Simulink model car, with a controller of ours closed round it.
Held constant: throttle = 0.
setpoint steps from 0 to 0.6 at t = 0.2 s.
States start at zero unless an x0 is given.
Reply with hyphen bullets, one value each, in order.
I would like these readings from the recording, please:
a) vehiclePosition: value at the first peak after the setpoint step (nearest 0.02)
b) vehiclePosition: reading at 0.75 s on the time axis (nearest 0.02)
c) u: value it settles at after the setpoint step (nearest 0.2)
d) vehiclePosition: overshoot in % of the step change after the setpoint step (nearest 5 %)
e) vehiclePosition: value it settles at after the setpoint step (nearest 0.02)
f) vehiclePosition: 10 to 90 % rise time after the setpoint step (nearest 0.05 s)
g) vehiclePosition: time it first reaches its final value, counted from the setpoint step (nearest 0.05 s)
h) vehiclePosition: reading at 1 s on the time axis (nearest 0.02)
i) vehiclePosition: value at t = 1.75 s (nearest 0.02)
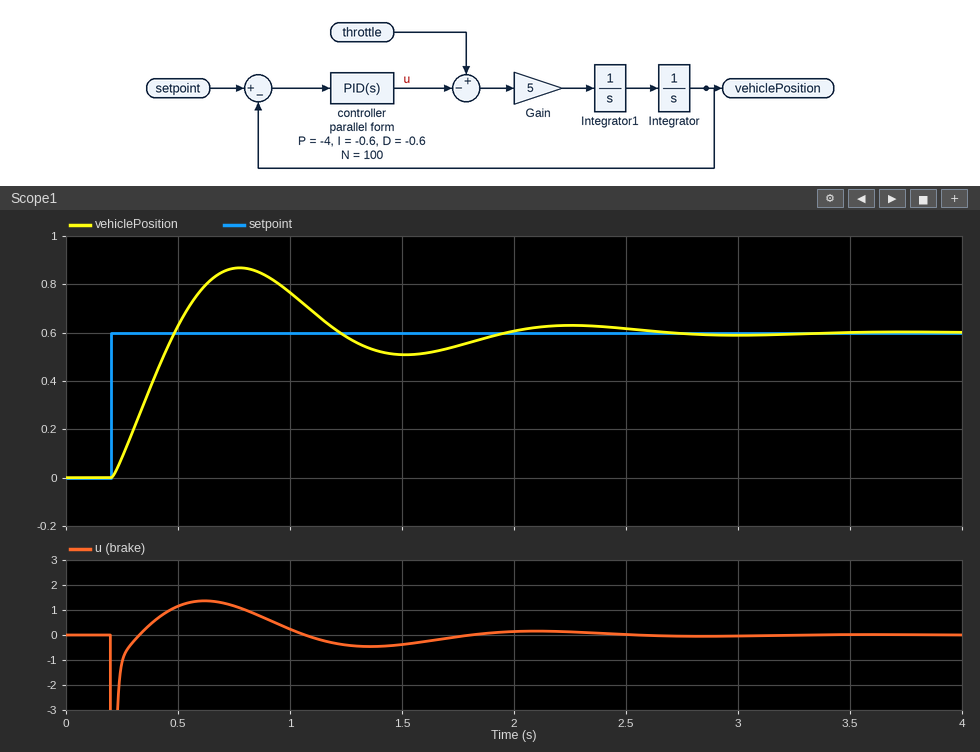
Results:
- 0.86
- 0.86
- 0.0
- 45 %
- 0.60
- 0.20 s
- 0.30 s
- 0.76
- 0.54
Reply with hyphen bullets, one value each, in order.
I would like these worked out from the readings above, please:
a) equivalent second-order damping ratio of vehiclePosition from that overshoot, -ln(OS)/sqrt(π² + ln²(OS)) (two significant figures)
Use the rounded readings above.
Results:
- 0.25
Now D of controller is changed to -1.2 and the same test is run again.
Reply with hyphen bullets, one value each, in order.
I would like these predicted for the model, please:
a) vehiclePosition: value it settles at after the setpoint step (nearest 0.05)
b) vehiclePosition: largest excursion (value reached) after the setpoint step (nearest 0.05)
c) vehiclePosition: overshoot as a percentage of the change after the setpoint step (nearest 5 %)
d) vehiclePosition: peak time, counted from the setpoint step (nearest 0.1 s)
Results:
- 0.60
- 0.75
- 25 %
- 0.5 s
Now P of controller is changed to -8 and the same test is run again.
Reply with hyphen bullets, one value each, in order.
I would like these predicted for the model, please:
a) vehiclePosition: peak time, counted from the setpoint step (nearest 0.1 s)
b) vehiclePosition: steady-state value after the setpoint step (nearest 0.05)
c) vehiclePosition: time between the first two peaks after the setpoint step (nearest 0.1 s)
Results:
- 0.4 s
- 0.60
- 1.0 s
